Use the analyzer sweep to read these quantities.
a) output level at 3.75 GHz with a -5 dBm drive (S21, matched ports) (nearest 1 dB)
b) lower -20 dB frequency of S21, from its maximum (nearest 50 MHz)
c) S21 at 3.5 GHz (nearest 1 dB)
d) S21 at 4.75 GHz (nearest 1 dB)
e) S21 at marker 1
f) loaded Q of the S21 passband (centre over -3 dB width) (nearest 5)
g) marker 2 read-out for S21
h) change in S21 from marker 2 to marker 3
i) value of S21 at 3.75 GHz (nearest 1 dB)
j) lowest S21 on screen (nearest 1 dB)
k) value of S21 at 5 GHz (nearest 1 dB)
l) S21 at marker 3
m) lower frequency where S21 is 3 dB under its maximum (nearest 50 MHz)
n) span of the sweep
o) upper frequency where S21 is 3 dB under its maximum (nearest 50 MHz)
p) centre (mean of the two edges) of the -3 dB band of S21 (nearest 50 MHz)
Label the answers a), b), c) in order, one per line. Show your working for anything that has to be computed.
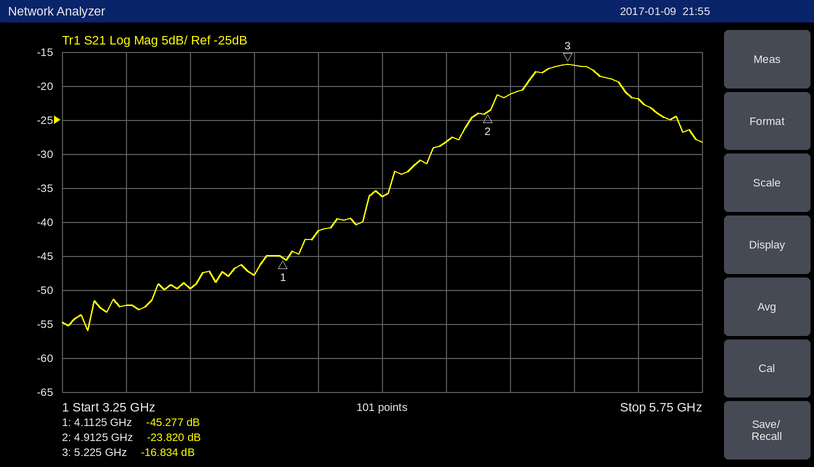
a) -5 dBm + (-50 dB) = -55 dBm
b) 4.45 GHz
c) -52 dB
d) -28 dB
e) -45.277 dB
f) 5.25 GHz / 400 MHz ≈ 13.1, so 15 to the nearest 5
g) -23.820 dB
h) -16.834 − (-23.82) = 6.986 dB
i) -50 dB
j) -56 dB
k) -21 dB
l) -16.834 dB
m) 5.05 GHz
n) 2.5 GHz
o) 5.45 GHz
p) 5.25 GHz
